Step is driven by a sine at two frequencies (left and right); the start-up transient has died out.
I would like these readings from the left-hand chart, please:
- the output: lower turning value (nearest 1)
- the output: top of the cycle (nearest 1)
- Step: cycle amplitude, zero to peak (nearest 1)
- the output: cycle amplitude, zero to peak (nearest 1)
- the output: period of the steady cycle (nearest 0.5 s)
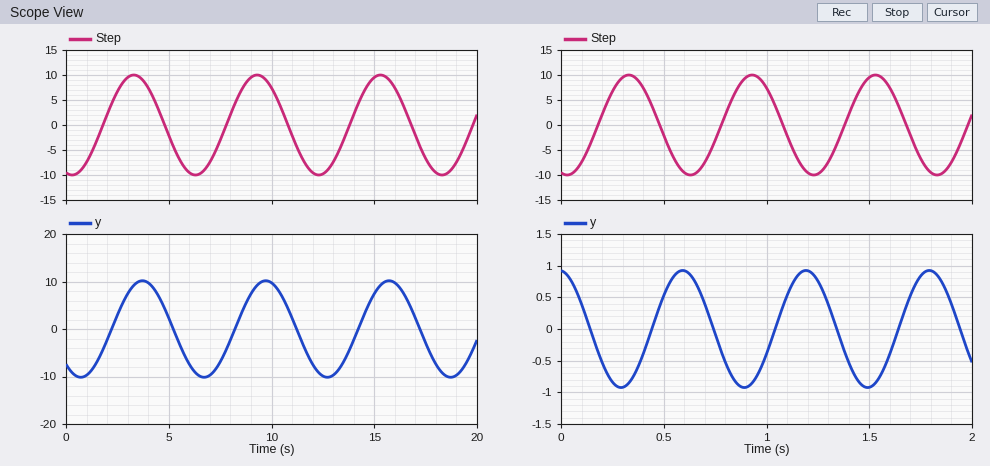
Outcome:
-10
10
10
10
6.0 s
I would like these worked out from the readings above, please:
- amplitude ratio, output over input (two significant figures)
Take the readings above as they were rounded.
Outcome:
1.0
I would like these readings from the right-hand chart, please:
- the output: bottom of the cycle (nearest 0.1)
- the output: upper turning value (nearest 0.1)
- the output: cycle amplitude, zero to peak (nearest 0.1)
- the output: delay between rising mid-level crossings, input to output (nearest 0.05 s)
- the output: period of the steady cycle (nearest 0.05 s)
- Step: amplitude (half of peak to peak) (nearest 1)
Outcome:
-0.9
0.9
0.9
0.25 s
0.60 s
10
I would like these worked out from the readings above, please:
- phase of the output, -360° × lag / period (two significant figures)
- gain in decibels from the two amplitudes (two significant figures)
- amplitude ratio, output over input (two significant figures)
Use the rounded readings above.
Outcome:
-150°
-21 dB
0.090
